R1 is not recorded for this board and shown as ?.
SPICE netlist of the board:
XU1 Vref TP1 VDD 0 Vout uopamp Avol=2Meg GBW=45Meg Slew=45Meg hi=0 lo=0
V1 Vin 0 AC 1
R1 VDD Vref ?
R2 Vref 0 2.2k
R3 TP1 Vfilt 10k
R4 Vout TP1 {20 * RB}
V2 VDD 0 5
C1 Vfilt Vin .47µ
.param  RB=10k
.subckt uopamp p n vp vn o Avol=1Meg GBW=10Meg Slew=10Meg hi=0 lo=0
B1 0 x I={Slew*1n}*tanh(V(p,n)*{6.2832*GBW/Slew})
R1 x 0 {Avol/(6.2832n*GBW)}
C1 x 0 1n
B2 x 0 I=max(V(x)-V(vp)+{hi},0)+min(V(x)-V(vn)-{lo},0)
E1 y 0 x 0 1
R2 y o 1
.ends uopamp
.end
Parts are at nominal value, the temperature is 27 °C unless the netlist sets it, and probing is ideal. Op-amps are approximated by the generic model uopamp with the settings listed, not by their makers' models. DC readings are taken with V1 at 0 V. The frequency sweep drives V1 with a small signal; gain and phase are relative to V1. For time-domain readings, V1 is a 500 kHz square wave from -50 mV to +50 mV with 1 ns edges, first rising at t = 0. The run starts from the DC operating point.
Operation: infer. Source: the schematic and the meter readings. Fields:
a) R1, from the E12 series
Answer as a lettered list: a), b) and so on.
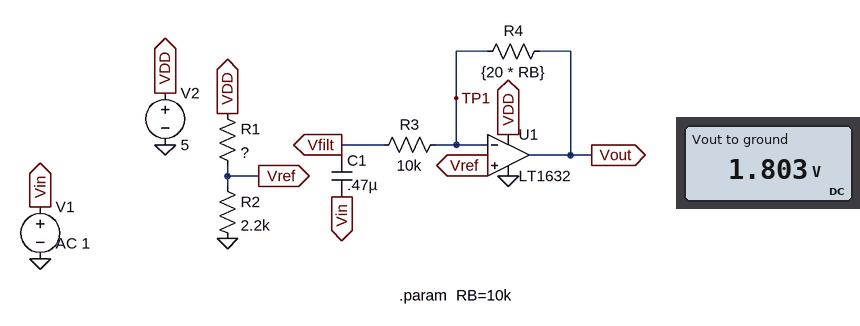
a) 3.9 kΩ
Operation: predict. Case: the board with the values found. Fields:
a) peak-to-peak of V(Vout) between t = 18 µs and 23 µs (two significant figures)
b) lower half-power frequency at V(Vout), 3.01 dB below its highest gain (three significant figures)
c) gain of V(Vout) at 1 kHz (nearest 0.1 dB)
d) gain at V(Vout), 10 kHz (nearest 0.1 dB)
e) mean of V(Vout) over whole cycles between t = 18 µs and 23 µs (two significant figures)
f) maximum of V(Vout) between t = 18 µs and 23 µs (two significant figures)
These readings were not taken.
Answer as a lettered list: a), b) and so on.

a) 1.8 V
b) 33.9 Hz
c) 26.0 dB
d) 26.0 dB
e) 890 mV
f) 1.8 V
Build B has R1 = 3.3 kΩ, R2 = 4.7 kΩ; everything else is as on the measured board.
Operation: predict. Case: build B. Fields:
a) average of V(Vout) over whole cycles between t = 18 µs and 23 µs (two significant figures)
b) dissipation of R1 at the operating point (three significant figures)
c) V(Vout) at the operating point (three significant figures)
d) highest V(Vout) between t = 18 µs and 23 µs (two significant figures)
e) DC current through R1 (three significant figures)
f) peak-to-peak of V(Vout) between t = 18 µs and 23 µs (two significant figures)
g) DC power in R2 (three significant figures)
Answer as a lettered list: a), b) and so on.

a) 1.9 V
b) 1.29 mW
c) 2.94 V
d) 2.9 V
e) 625 µA
f) 2.0 V
g) 1.84 mW
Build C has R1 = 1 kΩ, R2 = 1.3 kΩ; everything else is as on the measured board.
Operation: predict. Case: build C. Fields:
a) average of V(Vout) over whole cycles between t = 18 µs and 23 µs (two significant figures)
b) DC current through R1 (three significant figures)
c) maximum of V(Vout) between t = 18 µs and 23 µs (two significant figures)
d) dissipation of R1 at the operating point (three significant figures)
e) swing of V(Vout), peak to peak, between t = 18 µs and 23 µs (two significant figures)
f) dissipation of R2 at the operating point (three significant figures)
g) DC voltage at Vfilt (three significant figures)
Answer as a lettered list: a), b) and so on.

a) 1.8 V
b) 2.17 mA
c) 2.8 V
d) 4.73 mW
e) 2.0 V
f) 6.14 mW
g) 2.83 V
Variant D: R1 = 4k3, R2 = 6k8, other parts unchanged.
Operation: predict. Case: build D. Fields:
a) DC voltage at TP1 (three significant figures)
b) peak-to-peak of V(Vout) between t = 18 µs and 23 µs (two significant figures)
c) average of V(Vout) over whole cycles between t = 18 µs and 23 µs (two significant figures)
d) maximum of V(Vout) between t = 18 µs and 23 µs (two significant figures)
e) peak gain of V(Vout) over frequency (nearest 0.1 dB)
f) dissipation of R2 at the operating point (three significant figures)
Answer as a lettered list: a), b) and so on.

a) 3.06 V
b) 2.0 V
c) 2.1 V
d) 3.1 V
e) 26.0 dB
f) 1.38 mW
